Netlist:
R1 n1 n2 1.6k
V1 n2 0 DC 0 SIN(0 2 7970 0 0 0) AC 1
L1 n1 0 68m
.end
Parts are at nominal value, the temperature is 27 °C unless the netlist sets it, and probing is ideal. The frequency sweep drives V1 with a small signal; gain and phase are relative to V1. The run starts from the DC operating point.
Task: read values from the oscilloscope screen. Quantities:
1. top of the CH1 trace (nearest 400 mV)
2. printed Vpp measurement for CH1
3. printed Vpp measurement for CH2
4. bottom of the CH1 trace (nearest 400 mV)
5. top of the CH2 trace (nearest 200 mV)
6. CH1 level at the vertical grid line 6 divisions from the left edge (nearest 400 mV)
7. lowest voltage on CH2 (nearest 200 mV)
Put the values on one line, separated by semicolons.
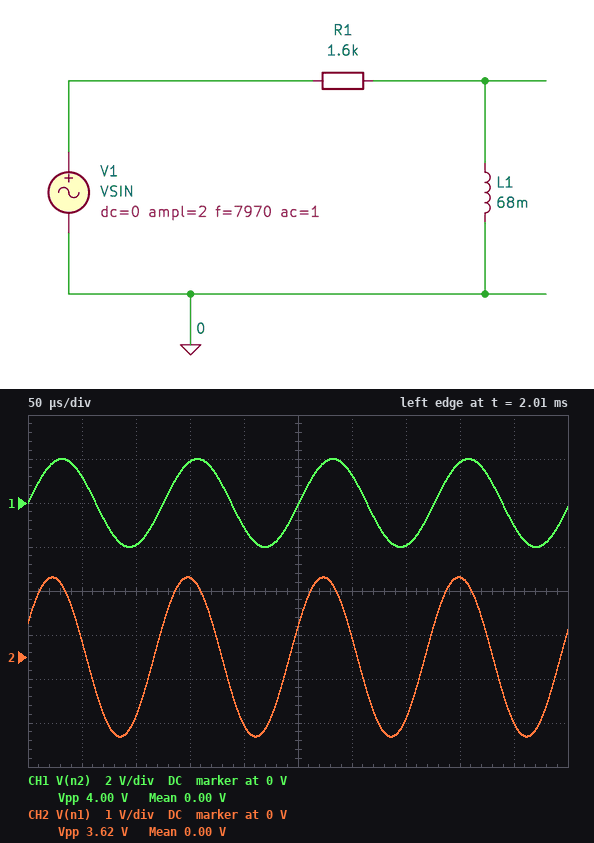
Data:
2.0 V; 4.00 V; 3.62 V; -2.0 V; 1.8 V; 1.2 V; -1.8 V
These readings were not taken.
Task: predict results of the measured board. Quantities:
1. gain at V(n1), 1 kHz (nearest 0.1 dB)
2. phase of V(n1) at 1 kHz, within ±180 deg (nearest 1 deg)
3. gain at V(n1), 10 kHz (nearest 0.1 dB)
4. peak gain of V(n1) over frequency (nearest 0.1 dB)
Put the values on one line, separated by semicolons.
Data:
-11.8 dB; 75 deg; -0.6 dB; 0 dB
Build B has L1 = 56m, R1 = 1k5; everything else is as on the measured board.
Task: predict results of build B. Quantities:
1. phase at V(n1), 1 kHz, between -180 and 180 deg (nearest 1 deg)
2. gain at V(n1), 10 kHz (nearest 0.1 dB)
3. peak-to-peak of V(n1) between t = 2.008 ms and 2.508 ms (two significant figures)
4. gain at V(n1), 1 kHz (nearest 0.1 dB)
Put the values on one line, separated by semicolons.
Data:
77 deg; -0.7 dB; 3.5 V; -12.8 dB
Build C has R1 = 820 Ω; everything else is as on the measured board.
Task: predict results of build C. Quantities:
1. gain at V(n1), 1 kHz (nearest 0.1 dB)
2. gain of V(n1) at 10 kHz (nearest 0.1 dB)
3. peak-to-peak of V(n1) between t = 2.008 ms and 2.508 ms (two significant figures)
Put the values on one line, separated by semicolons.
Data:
-6.7 dB; -0.2 dB; 3.9 V
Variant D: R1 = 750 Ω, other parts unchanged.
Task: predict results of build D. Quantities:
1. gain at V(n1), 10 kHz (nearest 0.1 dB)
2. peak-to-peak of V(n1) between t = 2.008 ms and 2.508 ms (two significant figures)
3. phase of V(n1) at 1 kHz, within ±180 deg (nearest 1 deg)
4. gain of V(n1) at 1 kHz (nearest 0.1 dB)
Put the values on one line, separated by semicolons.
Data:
-0.1 dB; 3.9 V; 60 deg; -6.1 dB
